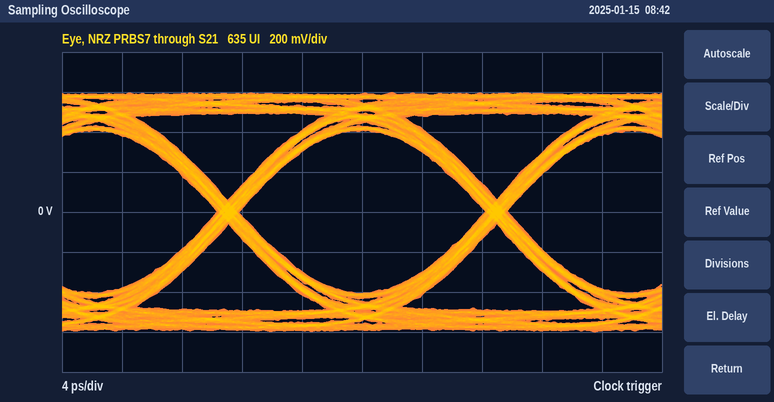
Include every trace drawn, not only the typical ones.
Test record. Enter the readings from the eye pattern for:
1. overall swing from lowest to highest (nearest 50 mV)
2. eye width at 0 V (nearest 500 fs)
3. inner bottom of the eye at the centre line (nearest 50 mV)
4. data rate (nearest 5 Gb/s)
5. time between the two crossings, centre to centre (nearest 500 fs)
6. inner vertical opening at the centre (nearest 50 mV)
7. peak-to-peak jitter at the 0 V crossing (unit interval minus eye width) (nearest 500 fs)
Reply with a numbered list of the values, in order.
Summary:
1. 1.20 V
2. 16.5 ps
3. -400 mV
4. 55 Gb/s
5. 18.0 ps
6. 800 mV
7. 1.5 ps
